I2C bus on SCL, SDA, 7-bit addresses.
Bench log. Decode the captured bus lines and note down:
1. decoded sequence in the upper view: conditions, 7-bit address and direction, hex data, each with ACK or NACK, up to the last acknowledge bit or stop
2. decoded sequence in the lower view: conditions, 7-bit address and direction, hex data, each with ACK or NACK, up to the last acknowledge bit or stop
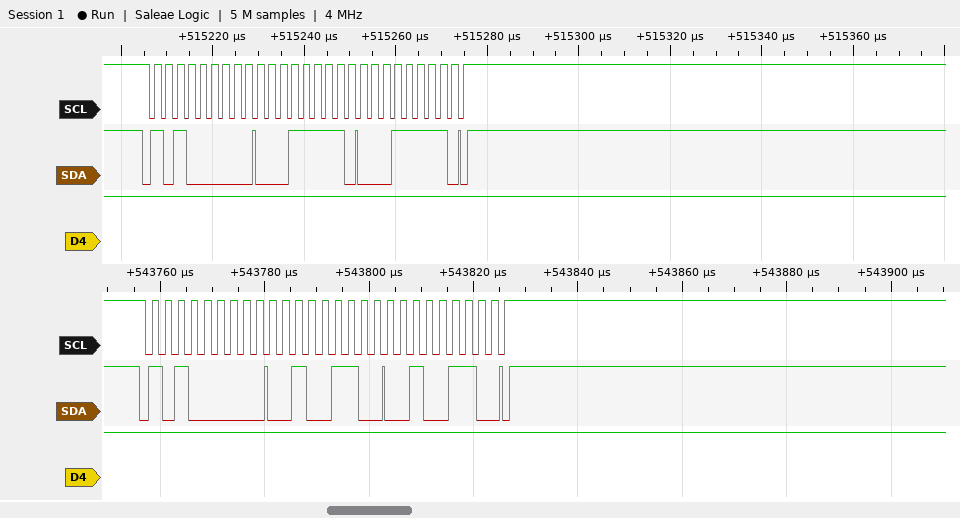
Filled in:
start, address 50 write ACK, 1F ACK, 1F ACK, stop
start, address 50 write ACK, 26 ACK, 26 ACK, stop
